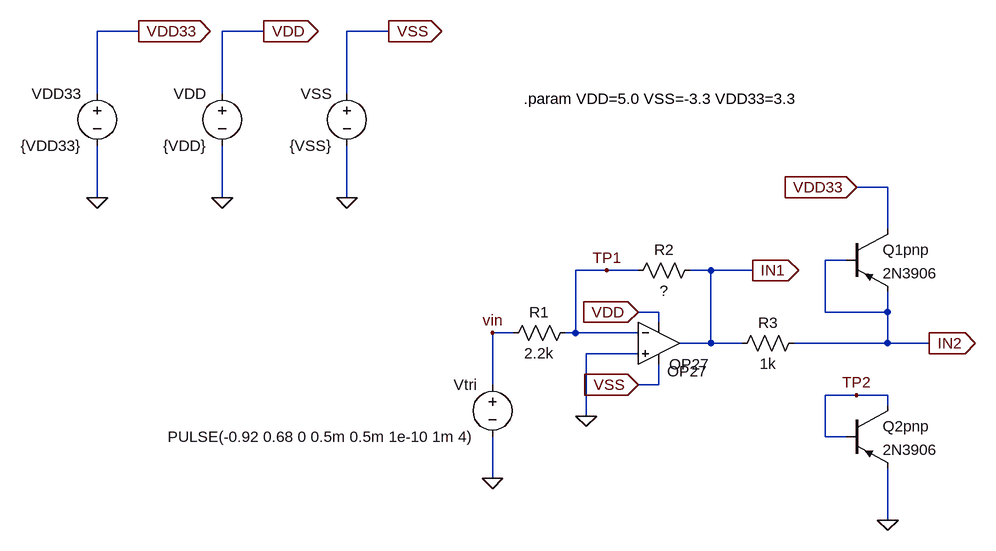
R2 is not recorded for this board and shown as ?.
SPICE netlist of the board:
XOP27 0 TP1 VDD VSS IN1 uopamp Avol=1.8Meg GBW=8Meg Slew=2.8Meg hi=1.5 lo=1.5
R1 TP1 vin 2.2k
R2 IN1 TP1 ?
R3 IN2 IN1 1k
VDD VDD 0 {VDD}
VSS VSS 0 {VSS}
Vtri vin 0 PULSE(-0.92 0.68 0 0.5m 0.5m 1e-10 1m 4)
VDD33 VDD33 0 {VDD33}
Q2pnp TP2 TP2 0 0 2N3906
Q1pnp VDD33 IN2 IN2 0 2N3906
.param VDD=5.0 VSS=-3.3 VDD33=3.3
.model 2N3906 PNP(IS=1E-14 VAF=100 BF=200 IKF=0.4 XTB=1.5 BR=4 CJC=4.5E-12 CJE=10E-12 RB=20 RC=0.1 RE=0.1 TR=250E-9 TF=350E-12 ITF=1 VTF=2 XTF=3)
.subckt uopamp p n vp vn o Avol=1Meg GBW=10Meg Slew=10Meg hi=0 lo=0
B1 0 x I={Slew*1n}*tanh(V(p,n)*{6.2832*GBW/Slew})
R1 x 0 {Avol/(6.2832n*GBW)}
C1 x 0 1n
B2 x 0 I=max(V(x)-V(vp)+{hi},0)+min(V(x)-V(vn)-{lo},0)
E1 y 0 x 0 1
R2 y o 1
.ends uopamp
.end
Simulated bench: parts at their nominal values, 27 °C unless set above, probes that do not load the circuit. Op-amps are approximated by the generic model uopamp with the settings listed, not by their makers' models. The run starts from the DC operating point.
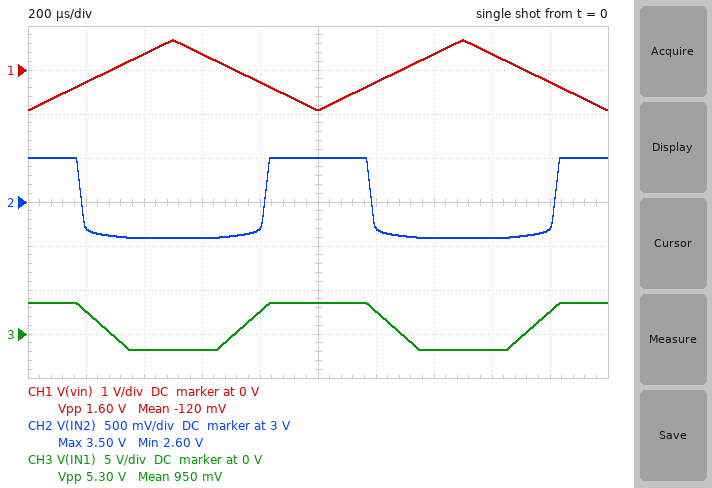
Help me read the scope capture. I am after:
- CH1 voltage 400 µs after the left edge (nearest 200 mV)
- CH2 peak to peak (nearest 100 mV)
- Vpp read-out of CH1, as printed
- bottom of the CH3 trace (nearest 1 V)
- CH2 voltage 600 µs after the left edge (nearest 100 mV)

400 mV
900 mV
1.60 V
-2 V
2.6 V
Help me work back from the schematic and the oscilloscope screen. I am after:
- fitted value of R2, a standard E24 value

20 kΩ
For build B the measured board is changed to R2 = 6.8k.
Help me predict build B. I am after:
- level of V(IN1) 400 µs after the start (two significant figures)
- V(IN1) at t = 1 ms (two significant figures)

-1.1 V
2.8 V
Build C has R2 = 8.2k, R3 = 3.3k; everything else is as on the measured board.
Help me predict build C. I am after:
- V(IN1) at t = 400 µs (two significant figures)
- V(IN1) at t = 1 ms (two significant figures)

-1.3 V
3.4 V
